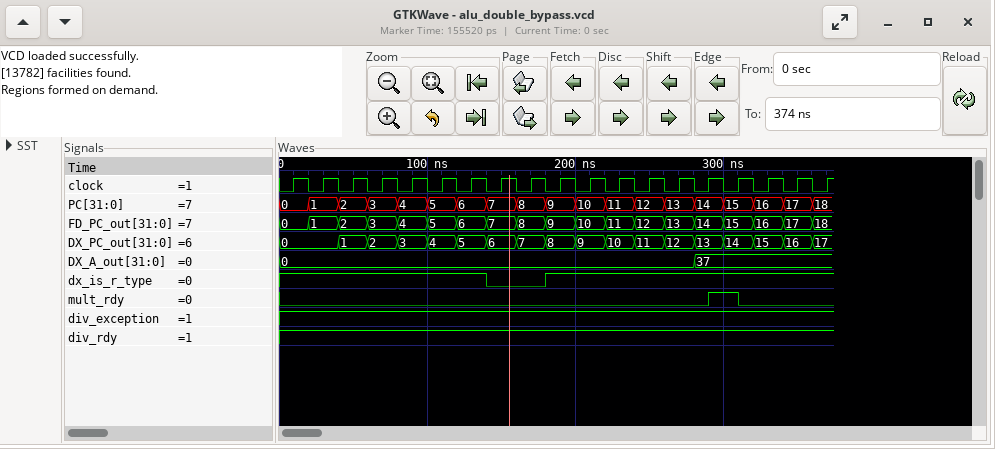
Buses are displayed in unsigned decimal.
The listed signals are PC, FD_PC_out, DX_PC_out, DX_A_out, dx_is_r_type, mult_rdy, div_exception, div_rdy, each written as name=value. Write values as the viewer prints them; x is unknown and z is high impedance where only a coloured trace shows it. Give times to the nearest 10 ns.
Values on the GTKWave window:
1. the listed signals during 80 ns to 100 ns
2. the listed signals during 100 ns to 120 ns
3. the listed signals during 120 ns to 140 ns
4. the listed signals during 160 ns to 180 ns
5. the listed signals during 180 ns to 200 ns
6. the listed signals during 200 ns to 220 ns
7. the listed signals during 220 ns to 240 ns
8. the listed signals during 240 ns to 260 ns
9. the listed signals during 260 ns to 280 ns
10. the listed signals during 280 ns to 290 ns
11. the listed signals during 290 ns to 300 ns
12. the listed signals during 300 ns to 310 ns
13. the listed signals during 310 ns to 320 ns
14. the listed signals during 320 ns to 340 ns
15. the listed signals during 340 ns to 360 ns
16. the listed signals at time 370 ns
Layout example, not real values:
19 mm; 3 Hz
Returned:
PC=4, FD_PC_out=4, DX_PC_out=3, DX_A_out=0, dx_is_r_type=1, mult_rdy=0, div_exception=1, div_rdy=1; PC=5, FD_PC_out=5, DX_PC_out=4, DX_A_out=0, dx_is_r_type=1, mult_rdy=0, div_exception=1, div_rdy=1; PC=6, FD_PC_out=6, DX_PC_out=5, DX_A_out=0, dx_is_r_type=1, mult_rdy=0, div_exception=1, div_rdy=1; PC=8, FD_PC_out=8, DX_PC_out=7, DX_A_out=0, dx_is_r_type=0, mult_rdy=0, div_exception=1, div_rdy=1; PC=9, FD_PC_out=9, DX_PC_out=8, DX_A_out=0, dx_is_r_type=1, mult_rdy=0, div_exception=1, div_rdy=1; PC=10, FD_PC_out=10, DX_PC_out=9, DX_A_out=0, dx_is_r_type=1, mult_rdy=0, div_exception=1, div_rdy=1; PC=11, FD_PC_out=11, DX_PC_out=10, DX_A_out=0, dx_is_r_type=1, mult_rdy=0, div_exception=1, div_rdy=1; PC=12, FD_PC_out=12, DX_PC_out=11, DX_A_out=0, dx_is_r_type=1, mult_rdy=0, div_exception=1, div_rdy=1; PC=13, FD_PC_out=13, DX_PC_out=12, DX_A_out=0, dx_is_r_type=1, mult_rdy=0, div_exception=1, div_rdy=1; PC=14, FD_PC_out=14, DX_PC_out=13, DX_A_out=37, dx_is_r_type=1, mult_rdy=0, div_exception=1, div_rdy=1; PC=14, FD_PC_out=14, DX_PC_out=13, DX_A_out=37, dx_is_r_type=1, mult_rdy=1, div_exception=1, div_rdy=1; PC=15, FD_PC_out=15, DX_PC_out=14, DX_A_out=37, dx_is_r_type=1, mult_rdy=1, div_exception=1, div_rdy=1; PC=15, FD_PC_out=15, DX_PC_out=14, DX_A_out=37, dx_is_r_type=1, mult_rdy=0, div_exception=1, div_rdy=1; PC=16, FD_PC_out=16, DX_PC_out=15, DX_A_out=37, dx_is_r_type=1, mult_rdy=0, div_exception=1, div_rdy=1; PC=17, FD_PC_out=17, DX_PC_out=16, DX_A_out=37, dx_is_r_type=1, mult_rdy=0, div_exception=1, div_rdy=1; PC=18, FD_PC_out=18, DX_PC_out=17, DX_A_out=37, dx_is_r_type=1, mult_rdy=0, div_exception=1, div_rdy=1
